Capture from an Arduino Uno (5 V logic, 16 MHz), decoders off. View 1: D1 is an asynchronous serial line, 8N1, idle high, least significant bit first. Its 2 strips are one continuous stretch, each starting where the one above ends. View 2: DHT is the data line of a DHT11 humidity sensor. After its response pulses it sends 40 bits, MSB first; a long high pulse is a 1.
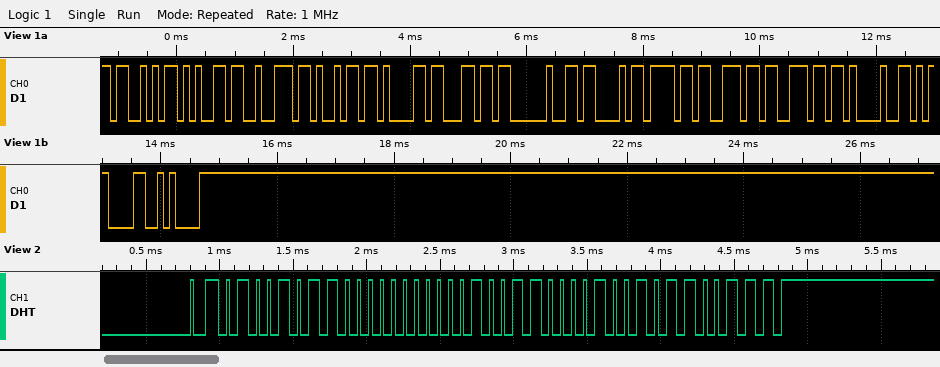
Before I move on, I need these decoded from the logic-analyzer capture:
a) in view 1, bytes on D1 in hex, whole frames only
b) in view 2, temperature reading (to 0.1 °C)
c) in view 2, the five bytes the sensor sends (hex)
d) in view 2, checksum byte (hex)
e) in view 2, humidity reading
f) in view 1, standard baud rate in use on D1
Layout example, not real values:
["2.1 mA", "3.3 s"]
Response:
["53 65 72 69 61 6C 20 43 6F 6E 6E 21 0D 0A", "19.9 °C", "4B 00 13 09 67", "0x67", "75 %", "9600 baud"]
